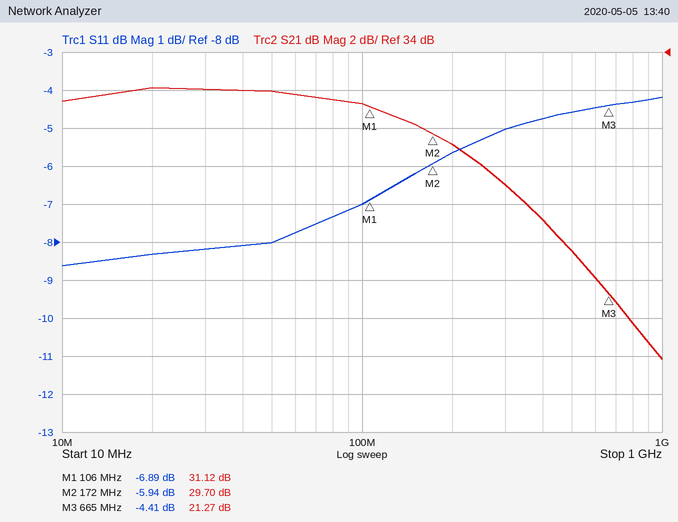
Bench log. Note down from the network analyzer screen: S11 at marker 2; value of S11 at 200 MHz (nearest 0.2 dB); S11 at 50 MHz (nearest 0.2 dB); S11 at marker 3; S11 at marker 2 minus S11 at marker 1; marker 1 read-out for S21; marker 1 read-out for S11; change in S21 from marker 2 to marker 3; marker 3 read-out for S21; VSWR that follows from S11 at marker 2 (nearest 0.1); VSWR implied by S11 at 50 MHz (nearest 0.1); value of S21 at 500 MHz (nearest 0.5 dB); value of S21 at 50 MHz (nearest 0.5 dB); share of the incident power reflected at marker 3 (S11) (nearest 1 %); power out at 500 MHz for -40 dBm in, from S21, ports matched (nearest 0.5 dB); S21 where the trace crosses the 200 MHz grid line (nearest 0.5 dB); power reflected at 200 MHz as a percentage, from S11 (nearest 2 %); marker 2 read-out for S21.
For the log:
-5.94 dB
-5.6 dB
-8.0 dB
-4.41 dB
0.95 dB
31.12 dB
-6.89 dB
-8.43 dB
21.27 dB
3.0
2.3
23.5 dB
32.0 dB
36 %
-16.5 dBm
29.0 dB
28 %
29.70 dB
